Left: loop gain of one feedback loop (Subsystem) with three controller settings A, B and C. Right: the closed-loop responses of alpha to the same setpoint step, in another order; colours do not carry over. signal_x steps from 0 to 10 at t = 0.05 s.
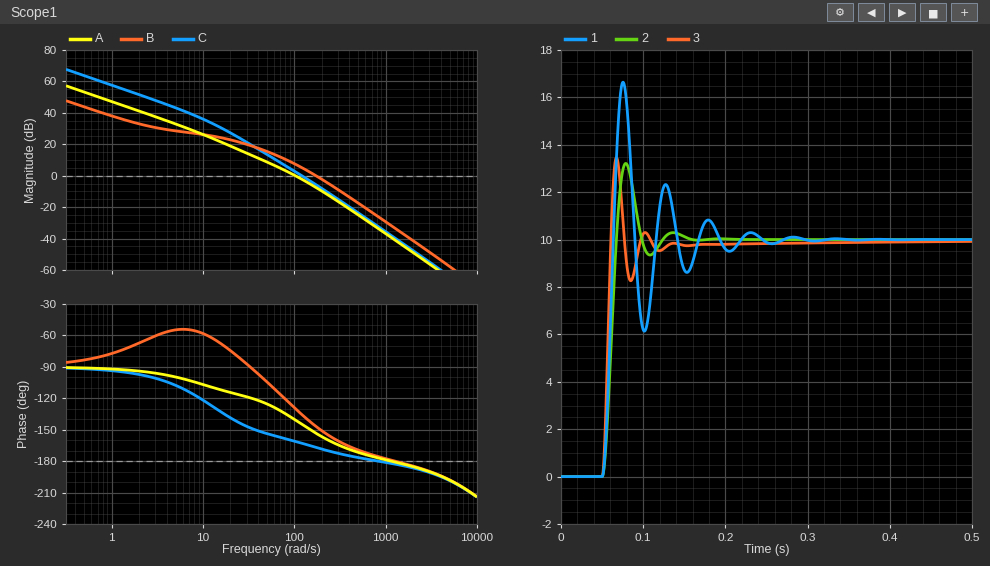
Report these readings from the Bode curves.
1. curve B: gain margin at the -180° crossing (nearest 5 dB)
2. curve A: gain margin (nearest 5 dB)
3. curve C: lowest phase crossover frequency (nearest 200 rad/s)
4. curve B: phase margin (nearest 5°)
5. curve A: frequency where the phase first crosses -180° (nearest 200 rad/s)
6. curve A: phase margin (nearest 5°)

35 dB
40 dB
800 rad/s
35°
1200 rad/s
40°
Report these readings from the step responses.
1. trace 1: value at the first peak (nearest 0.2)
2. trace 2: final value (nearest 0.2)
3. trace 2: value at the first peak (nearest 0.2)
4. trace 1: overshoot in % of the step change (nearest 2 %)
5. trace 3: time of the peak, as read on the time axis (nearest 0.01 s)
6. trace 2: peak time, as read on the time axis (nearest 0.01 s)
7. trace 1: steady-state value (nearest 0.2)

16.6
10.0
13.2
66 %
0.07 s
0.08 s
10.0
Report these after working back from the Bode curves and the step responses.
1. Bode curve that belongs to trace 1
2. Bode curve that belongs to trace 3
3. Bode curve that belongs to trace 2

C
B
A
